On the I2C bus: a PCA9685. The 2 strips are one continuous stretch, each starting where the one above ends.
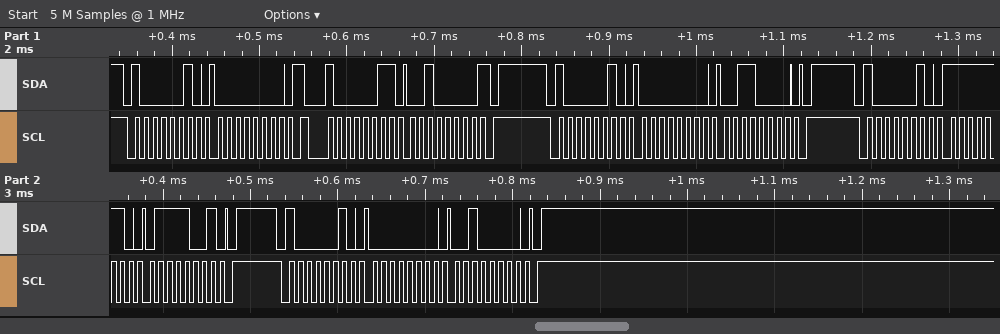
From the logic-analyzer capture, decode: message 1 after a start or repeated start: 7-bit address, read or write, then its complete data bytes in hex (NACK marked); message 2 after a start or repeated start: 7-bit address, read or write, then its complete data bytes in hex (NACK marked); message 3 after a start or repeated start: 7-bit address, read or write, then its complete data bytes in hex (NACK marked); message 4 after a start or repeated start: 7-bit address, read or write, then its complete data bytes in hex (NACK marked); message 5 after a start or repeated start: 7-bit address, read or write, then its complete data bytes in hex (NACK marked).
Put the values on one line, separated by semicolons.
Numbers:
0x41 write: 00; 0x41 read: 20 NACK; 0x41 write: 00 30; 0x41 write: FE 79; 0x41 write: 00 20
